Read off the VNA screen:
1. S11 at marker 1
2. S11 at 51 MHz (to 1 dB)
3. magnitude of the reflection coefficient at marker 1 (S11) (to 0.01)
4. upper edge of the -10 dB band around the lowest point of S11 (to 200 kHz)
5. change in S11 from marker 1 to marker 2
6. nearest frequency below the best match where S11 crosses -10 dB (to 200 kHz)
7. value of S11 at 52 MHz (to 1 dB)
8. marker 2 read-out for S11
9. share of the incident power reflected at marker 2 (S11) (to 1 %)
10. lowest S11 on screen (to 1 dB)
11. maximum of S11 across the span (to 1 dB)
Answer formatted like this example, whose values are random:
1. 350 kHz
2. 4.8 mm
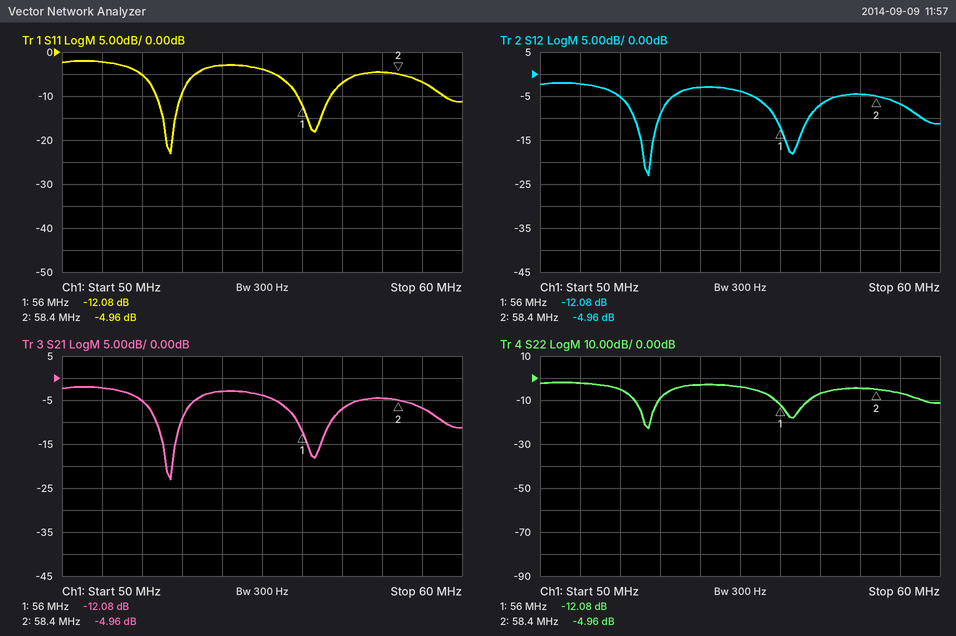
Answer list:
1. -12.08 dB
2. -2 dB
3. 0.25
4. 53.0 MHz
5. 7.12 dB
6. 52.4 MHz
7. -5 dB
8. -4.96 dB
9. 32 %
10. -23 dB
11. -2 dB
